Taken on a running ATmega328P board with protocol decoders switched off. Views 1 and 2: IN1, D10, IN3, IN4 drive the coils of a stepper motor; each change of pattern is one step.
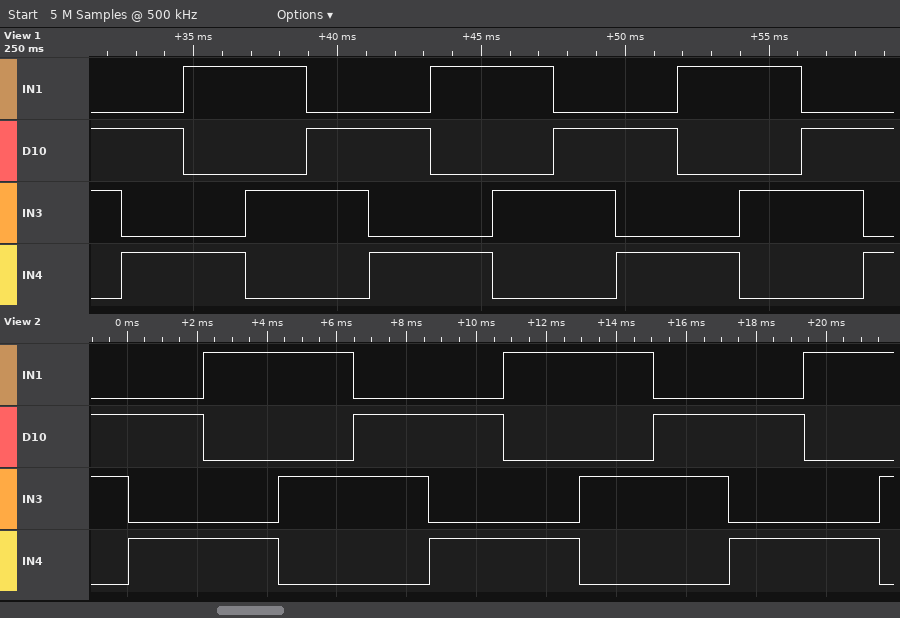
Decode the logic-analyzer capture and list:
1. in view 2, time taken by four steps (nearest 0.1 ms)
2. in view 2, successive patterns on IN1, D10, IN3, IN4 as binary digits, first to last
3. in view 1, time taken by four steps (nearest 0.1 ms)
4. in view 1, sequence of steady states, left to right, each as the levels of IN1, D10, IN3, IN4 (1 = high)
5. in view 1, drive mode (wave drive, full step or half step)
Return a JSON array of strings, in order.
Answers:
["8.6 ms", "0110 0101 1001 1010 0110 0101 1001 1010 0110 0101 1001 1010", "8.6 ms", "0110 0101 1001 1010 0110 0101 1001 1010 0110 0101 1001 1010 0110 0101", "full step"]
